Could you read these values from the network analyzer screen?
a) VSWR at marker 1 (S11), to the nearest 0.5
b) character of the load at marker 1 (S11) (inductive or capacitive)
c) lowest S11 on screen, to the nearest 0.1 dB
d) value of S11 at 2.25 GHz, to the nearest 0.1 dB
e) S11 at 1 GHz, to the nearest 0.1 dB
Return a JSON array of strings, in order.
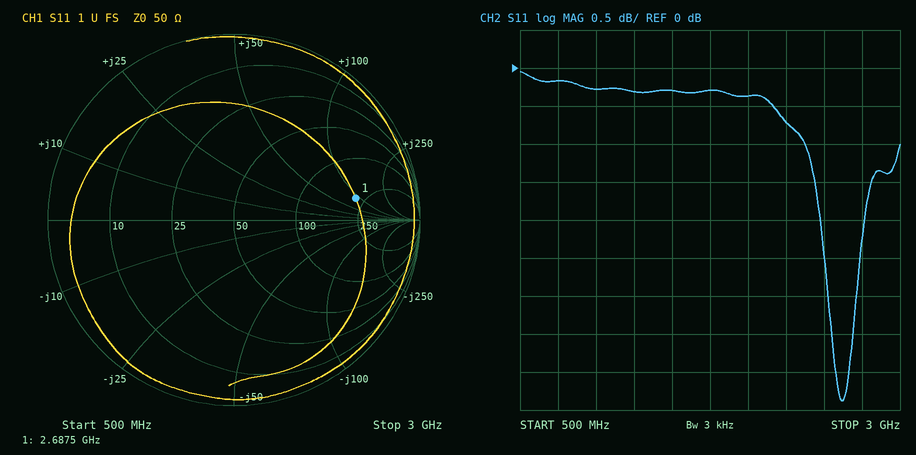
["5.0", "inductive", "-4.4 dB", "-0.7 dB", "-0.3 dB"]
